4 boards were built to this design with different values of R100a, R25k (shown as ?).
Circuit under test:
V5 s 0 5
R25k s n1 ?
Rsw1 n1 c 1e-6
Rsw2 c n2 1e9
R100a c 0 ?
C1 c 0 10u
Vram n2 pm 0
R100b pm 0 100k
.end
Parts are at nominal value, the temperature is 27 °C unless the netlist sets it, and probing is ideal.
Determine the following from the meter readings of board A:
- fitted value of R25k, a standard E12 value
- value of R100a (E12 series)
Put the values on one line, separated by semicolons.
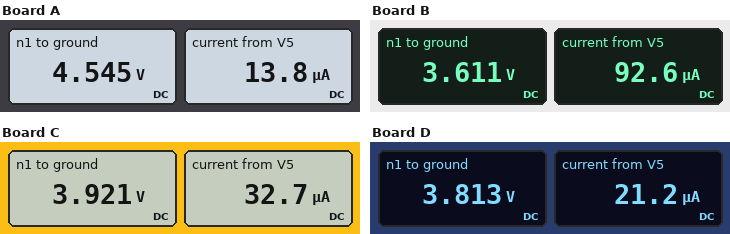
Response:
33 kΩ; 330 kΩ
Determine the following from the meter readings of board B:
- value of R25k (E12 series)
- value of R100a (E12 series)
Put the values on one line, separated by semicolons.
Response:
15 kΩ; 39 kΩ
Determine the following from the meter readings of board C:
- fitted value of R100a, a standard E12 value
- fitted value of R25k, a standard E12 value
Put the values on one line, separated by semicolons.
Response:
120 kΩ; 33 kΩ
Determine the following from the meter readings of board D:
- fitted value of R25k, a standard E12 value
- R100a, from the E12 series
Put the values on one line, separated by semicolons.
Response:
56 kΩ; 180 kΩ
